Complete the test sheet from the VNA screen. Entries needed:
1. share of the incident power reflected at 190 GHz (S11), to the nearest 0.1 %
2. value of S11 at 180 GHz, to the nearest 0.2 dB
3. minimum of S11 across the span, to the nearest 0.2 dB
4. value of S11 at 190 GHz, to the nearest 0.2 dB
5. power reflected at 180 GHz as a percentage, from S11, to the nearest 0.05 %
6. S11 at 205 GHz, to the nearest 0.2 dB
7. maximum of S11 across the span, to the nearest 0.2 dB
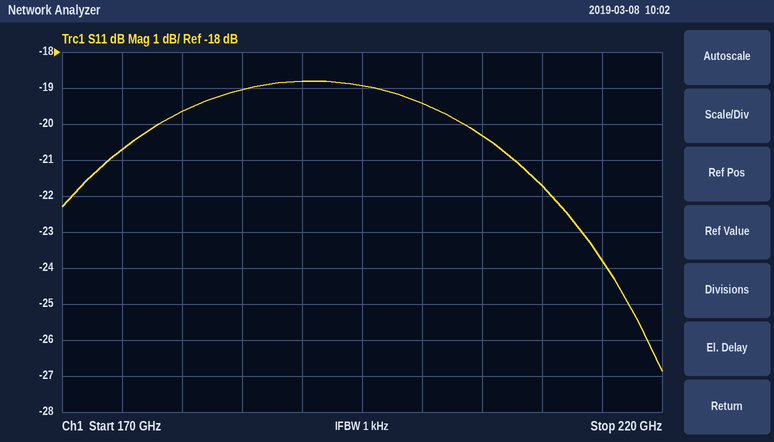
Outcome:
1.3 %
-19.6 dB
-26.8 dB
-18.8 dB
1.10 %
-20.4 dB
-18.8 dB
